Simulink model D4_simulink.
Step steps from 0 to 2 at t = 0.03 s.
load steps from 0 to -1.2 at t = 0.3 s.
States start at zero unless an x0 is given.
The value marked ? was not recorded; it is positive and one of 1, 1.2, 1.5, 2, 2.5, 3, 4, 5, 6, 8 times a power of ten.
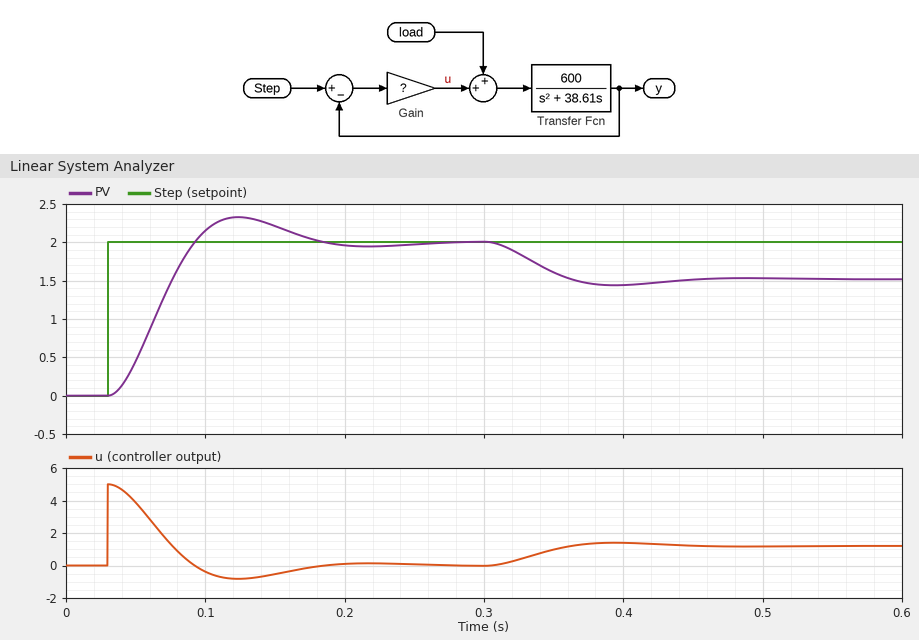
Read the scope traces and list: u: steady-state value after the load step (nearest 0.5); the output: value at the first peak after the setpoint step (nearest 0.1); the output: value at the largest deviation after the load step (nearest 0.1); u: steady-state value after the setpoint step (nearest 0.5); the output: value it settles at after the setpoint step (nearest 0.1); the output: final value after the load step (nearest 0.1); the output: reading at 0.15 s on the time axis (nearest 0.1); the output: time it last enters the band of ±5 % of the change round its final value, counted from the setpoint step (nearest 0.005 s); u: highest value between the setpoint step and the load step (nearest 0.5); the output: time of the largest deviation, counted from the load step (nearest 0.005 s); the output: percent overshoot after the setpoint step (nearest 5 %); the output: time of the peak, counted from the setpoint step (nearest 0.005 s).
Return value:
1.0
2.3
1.4
0.0
2.0
1.5
2.2
0.135 s
5.0
0.095 s
15 %
0.095 s
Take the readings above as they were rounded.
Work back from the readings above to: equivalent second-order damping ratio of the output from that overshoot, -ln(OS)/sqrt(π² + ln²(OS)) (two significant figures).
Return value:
0.52
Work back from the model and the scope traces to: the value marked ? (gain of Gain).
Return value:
2.5
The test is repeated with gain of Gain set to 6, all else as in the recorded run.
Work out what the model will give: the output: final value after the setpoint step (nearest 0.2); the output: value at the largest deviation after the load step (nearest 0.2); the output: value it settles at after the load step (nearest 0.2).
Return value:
2.0
1.8
1.8
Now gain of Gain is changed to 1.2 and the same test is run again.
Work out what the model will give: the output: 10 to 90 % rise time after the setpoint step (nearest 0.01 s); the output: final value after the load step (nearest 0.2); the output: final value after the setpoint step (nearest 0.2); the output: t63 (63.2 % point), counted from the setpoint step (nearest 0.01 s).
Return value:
0.08 s
1.0
2.0
0.07 s
